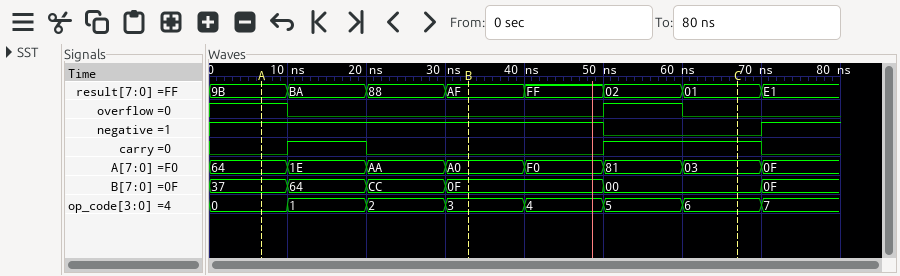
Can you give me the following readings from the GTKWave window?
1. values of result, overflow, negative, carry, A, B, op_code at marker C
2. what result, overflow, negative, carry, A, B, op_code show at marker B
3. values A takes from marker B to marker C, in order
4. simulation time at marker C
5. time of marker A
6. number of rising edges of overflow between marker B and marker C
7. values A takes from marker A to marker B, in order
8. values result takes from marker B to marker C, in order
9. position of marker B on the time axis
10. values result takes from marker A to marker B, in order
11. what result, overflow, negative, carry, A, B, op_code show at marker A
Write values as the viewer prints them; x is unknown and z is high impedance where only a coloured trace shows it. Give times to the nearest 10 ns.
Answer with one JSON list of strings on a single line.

["result=01, overflow=0, negative=0, carry=1, A=03, B=00, op_code=6", "result=AF, overflow=0, negative=1, carry=0, A=A0, B=0F, op_code=3", "A0, F0, 81, 03", "70 ns", "10 ns", "1", "64, 1E, AA, A0", "AF, FF, 02, 01", "30 ns", "9B, BA, 88, AF", "result=9B, overflow=1, negative=1, carry=0, A=64, B=37, op_code=0"]
